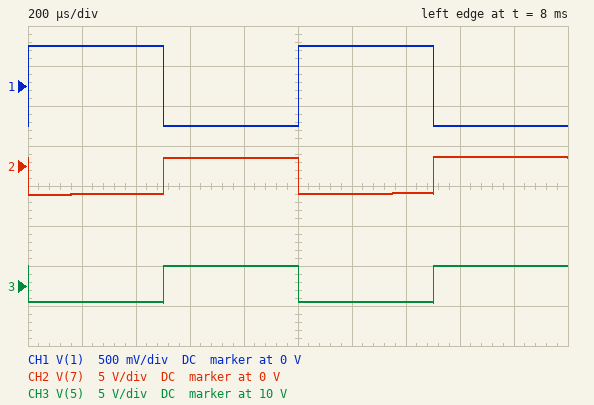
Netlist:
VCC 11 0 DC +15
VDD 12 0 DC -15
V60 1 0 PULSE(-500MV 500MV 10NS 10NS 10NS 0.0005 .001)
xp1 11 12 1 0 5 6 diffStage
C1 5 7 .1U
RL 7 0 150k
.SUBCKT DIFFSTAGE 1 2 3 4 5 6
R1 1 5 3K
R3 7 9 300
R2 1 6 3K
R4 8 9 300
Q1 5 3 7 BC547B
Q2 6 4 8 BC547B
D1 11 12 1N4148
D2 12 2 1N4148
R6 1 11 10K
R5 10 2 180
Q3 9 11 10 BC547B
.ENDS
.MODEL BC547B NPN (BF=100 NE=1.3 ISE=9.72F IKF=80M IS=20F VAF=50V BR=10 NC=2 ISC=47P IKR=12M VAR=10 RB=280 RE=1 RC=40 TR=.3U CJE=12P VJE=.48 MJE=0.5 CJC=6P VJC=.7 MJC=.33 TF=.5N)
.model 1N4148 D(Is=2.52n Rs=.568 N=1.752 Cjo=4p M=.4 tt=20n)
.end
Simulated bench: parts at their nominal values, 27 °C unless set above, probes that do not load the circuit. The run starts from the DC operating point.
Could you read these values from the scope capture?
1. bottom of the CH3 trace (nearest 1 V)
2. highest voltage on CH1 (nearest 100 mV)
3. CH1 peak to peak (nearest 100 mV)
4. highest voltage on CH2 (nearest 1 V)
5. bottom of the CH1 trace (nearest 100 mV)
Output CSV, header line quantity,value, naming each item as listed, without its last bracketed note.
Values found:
quantity,value
bottom of the CH3 trace,8 V
highest voltage on CH1,500 mV
CH1 peak to peak,1.0 V
highest voltage on CH2,1 V
bottom of the CH1 trace,-500 mV
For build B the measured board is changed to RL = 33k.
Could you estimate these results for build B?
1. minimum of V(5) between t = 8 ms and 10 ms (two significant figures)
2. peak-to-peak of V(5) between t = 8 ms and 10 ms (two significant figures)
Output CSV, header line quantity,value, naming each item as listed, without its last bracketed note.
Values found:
quantity,value
minimum of V(5) between t = 8 ms and 10 ms,8.0 V
peak-to-peak of V(5) between t = 8 ms and 10 ms,4.3 V
